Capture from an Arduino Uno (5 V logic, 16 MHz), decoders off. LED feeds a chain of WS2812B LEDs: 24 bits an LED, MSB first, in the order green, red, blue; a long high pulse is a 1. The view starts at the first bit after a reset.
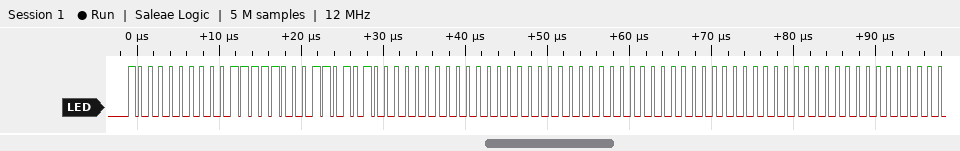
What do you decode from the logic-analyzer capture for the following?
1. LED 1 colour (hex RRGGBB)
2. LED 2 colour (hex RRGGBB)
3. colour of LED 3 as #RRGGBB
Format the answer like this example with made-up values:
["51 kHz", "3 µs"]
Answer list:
["#3E8035", "#000000", "#000000"]
